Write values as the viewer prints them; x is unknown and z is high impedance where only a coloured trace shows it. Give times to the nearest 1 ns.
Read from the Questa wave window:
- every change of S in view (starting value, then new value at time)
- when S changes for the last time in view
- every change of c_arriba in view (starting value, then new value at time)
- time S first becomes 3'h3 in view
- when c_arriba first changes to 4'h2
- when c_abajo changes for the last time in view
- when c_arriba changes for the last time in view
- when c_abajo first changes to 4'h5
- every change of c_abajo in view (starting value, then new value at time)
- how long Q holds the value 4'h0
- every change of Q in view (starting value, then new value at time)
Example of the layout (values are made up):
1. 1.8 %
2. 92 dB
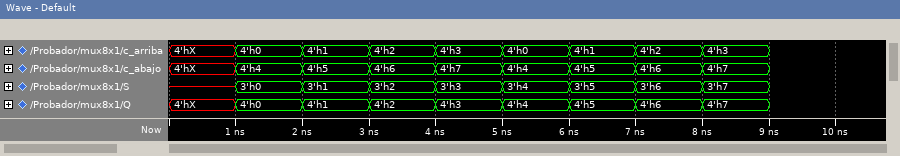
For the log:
1. x, 3'h0 at 1 ns, 3'h1 at 2 ns, 3'h2 at 3 ns, 3'h3 at 4 ns, 3'h4 at 5 ns, 3'h5 at 6 ns, 3'h6 at 7 ns, 3'h7 at 8 ns
2. 8 ns
3. 4'hX, 4'h0 at 1 ns, 4'h1 at 2 ns, 4'h2 at 3 ns, 4'h3 at 4 ns, 4'h0 at 5 ns, 4'h1 at 6 ns, 4'h2 at 7 ns, 4'h3 at 8 ns
4. 4 ns
5. 3 ns
6. 8 ns
7. 8 ns
8. 2 ns
9. 4'hX, 4'h4 at 1 ns, 4'h5 at 2 ns, 4'h6 at 3 ns, 4'h7 at 4 ns, 4'h4 at 5 ns, 4'h5 at 6 ns, 4'h6 at 7 ns, 4'h7 at 8 ns
10. 1 ns
11. 4'hX, 4'h0 at 1 ns, 4'h1 at 2 ns, 4'h2 at 3 ns, 4'h3 at 4 ns, 4'h4 at 5 ns, 4'h5 at 6 ns, 4'h6 at 7 ns, 4'h7 at 8 ns
